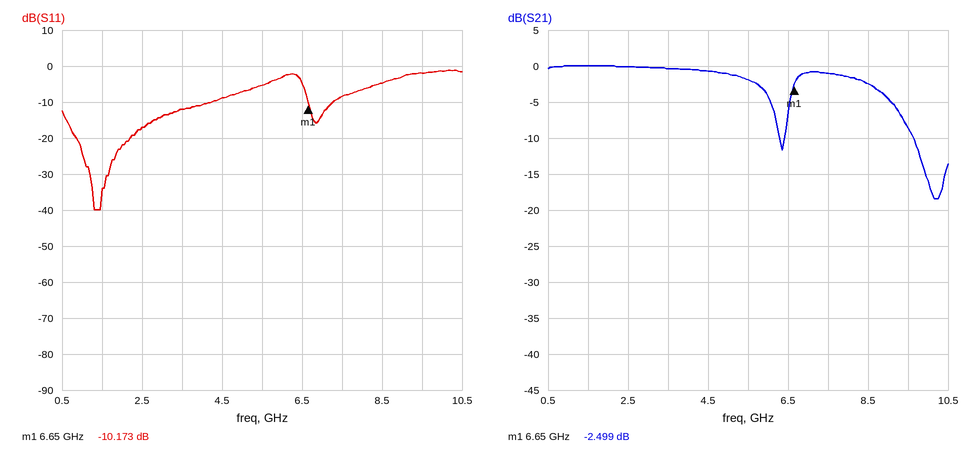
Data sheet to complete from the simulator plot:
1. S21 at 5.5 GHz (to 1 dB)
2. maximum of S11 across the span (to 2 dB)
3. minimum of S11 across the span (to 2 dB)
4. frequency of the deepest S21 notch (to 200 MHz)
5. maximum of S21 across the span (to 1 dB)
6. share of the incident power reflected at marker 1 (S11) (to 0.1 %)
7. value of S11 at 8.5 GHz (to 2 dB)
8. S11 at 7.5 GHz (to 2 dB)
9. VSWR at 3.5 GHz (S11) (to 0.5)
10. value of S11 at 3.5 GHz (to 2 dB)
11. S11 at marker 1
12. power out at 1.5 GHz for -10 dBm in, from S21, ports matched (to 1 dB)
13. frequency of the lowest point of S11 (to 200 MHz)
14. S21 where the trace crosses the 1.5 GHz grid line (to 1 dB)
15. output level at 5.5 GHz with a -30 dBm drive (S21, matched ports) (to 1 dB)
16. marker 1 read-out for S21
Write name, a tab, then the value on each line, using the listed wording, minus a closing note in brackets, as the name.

S21 at 5.5 GHz	-2 dB
maximum of S11 across the span	-2 dB
minimum of S11 across the span	-40 dB
frequency of the deepest S21 notch	10.2 GHz
maximum of S21 across the span	0 dB
share of the incident power reflected at marker 1 (S11)	9.6 %
value of S11 at 8.5 GHz	-4 dB
S11 at 7.5 GHz	-8 dB
VSWR at 3.5 GHz (S11)	1.5
value of S11 at 3.5 GHz	-12 dB
S11 at marker 1	-10.173 dB
power out at 1.5 GHz for -10 dBm in, from S21, ports matched	-10 dBm
frequency of the lowest point of S11	1.4 GHz
S21 where the trace crosses the 1.5 GHz grid line	0 dB
output level at 5.5 GHz with a -30 dBm drive (S21, matched ports)	-32 dBm
marker 1 read-out for S21	-2.499 dB
